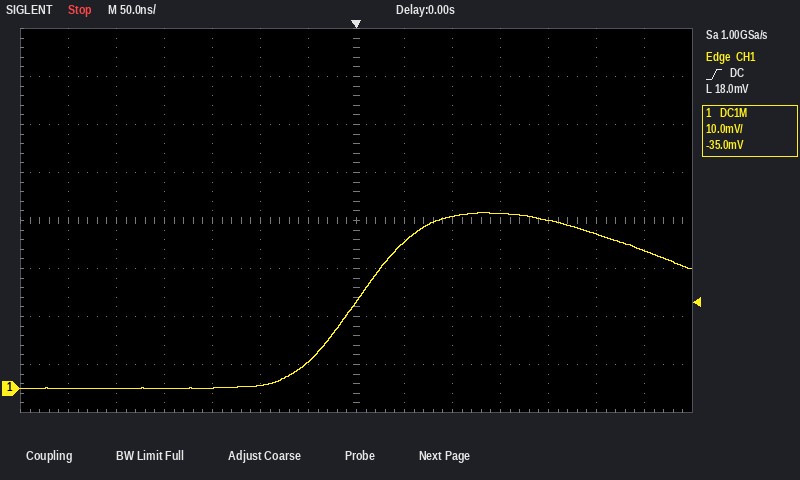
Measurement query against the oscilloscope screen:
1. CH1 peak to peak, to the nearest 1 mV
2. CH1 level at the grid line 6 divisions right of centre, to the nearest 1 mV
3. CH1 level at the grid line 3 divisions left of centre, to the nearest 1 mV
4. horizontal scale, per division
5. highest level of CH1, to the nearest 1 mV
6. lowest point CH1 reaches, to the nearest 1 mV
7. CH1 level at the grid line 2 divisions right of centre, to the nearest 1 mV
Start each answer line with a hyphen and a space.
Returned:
- 37 mV
- 29 mV
- 0 mV
- 50 ns
- 37 mV
- 0 mV
- 36 mV
